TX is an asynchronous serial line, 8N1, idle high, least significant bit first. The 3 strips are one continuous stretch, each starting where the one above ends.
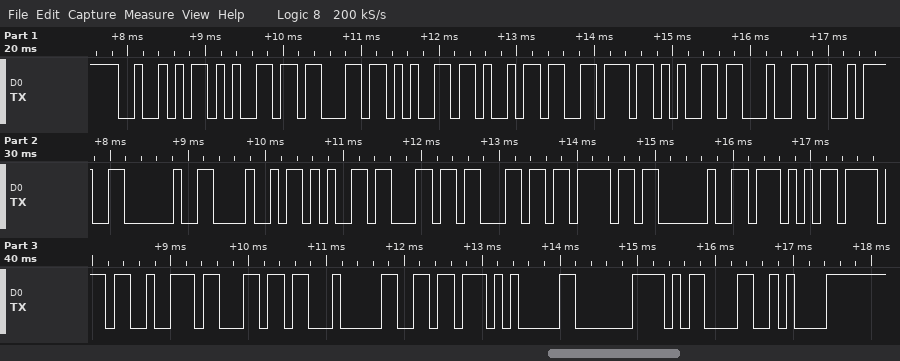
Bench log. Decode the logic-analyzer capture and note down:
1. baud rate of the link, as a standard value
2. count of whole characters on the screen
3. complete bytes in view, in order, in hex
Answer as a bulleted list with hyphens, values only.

- 9600 baud
- 26
- 52 65 63 65 69 76 65 64 3A 20 48 65 6C 6C 6F 20 57 6F 72 6C 04 B6 05 C0 0D 0A
